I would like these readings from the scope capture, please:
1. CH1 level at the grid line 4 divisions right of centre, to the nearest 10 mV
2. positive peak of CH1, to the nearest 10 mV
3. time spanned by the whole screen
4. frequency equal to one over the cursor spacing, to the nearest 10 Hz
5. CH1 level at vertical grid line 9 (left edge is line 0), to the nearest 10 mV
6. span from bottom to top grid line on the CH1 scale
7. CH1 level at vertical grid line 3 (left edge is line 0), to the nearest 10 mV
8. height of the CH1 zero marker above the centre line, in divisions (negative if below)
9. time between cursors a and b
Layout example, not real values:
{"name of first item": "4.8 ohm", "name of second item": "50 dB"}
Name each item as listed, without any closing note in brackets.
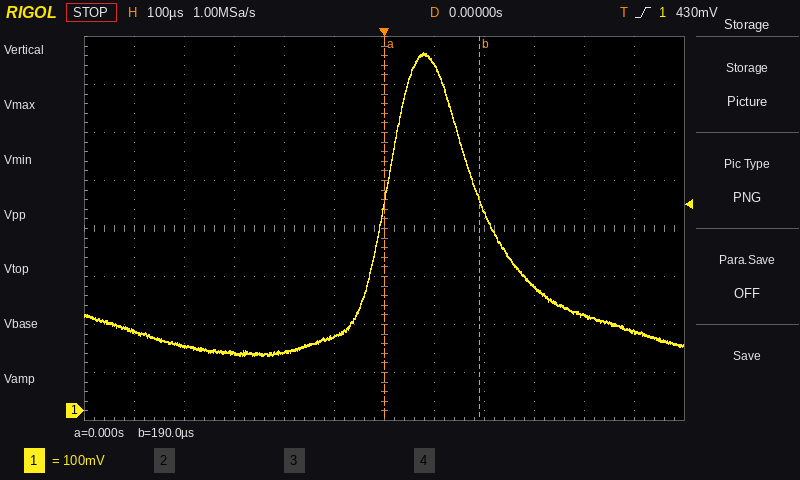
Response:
{"CH1 level at the grid line 4 divisions right of centre, to the nearest 10 mV": "200 mV", "positive peak of CH1, to the nearest 10 mV": "750 mV", "time spanned by the whole screen": "1.2 ms", "frequency equal to one over the cursor spacing, to the nearest 10 Hz": "5.26 kHz", "CH1 level at vertical grid line 9 (left edge is line 0), to the nearest 10 mV": "260 mV", "span from bottom to top grid line on the CH1 scale": "800 mV", "CH1 level at vertical grid line 3 (left edge is line 0), to the nearest 10 mV": "120 mV", "height of the CH1 zero marker above the centre line, in divisions": "-3.8 div", "time between cursors a and b": "190 µs"}
